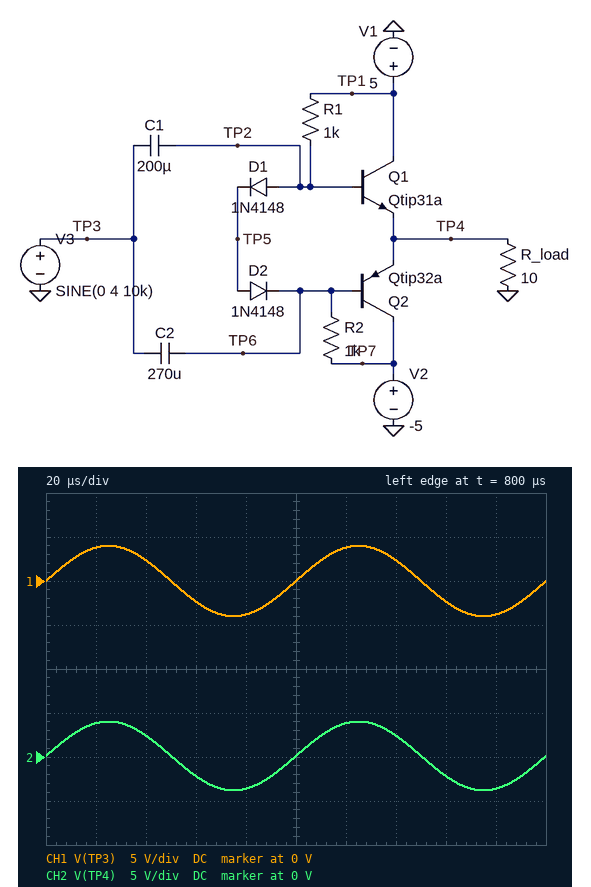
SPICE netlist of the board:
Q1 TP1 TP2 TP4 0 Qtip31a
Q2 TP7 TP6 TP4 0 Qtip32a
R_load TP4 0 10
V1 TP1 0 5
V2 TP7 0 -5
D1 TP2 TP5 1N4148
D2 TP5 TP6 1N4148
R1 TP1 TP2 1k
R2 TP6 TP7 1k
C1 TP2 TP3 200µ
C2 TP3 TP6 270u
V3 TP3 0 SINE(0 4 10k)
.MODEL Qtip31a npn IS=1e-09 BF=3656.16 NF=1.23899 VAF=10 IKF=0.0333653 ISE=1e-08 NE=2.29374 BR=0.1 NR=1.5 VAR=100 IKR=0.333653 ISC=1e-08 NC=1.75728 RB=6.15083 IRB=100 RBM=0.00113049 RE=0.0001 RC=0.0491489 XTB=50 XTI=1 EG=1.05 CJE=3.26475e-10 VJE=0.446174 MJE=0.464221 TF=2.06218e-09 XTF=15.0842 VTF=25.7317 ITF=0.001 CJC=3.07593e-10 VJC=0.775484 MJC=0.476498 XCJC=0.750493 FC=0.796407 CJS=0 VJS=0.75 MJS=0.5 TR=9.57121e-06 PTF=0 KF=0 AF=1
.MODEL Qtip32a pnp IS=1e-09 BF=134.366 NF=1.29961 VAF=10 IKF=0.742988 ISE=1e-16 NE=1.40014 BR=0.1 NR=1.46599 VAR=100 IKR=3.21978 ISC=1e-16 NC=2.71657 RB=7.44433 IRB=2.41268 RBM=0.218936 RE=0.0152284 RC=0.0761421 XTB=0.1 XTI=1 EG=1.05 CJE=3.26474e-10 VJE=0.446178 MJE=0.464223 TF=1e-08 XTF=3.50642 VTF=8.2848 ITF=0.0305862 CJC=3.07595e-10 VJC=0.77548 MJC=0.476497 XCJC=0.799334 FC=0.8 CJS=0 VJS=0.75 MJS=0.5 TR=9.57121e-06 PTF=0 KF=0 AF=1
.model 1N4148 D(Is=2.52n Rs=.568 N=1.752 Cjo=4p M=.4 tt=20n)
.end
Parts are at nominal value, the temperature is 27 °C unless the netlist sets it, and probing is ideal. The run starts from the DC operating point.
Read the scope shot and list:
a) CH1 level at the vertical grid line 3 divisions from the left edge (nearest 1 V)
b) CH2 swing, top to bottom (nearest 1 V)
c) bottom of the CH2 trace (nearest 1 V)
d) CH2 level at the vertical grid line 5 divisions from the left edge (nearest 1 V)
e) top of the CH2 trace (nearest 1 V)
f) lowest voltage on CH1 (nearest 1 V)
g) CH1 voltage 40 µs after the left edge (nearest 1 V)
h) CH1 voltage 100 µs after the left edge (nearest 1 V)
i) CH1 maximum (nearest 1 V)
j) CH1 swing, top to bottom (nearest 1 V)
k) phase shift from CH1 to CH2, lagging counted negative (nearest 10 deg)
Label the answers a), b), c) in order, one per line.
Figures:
a) -2 V
b) 8 V
c) -4 V
d) 0 V
e) 4 V
f) -4 V
g) 2 V
h) 0 V
i) 4 V
j) 8 V
k) 0 deg
